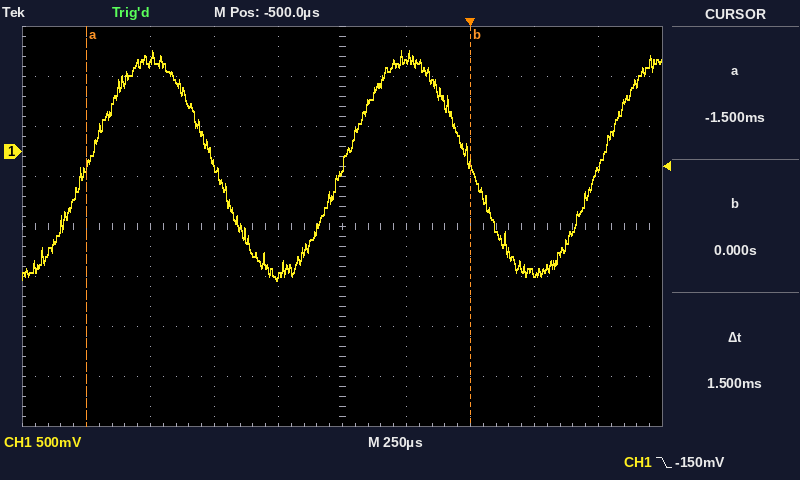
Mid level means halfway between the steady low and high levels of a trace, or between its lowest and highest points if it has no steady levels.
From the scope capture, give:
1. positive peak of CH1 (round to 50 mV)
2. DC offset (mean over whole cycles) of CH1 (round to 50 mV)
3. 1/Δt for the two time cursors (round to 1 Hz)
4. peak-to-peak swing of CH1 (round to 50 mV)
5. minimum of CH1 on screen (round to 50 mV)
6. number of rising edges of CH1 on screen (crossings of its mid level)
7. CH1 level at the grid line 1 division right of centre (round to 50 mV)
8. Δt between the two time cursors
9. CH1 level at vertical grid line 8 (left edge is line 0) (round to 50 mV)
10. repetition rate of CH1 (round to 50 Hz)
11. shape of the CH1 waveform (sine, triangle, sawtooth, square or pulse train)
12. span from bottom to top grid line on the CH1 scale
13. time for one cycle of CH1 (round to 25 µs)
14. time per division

1.00 V
-150 mV
667 Hz
2.30 V
-1.30 V
3
950 mV
1.5 ms
-1.20 V
1.00 kHz
sine
4 V
1.000 ms
250 µs
